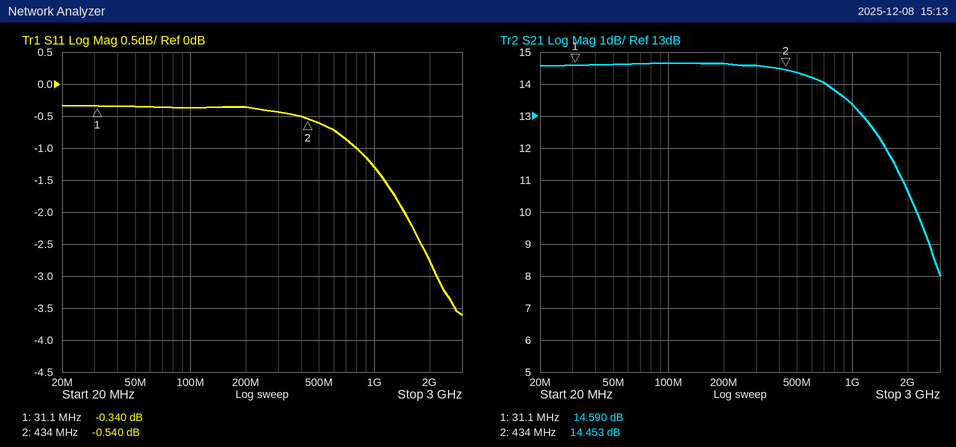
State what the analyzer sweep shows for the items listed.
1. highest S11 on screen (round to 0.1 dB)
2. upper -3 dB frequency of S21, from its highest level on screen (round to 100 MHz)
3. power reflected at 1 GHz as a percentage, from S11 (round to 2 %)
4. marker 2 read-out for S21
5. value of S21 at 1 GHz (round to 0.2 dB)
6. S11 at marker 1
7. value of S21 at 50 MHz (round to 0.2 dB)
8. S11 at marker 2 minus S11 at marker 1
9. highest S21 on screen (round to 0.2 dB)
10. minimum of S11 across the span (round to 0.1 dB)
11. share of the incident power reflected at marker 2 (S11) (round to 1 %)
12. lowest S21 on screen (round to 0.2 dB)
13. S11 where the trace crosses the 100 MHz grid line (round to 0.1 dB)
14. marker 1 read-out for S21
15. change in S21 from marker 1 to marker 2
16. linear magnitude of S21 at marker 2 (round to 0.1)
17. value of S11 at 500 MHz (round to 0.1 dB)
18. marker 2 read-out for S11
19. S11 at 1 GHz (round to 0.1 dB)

-0.3 dB
1.6 GHz
74 %
14.453 dB
13.4 dB
-0.340 dB
14.6 dB
-0.200 dB
14.6 dB
-3.6 dB
88 %
8.0 dB
-0.4 dB
14.590 dB
-0.137 dB
5.3
-0.6 dB
-0.540 dB
-1.3 dB
